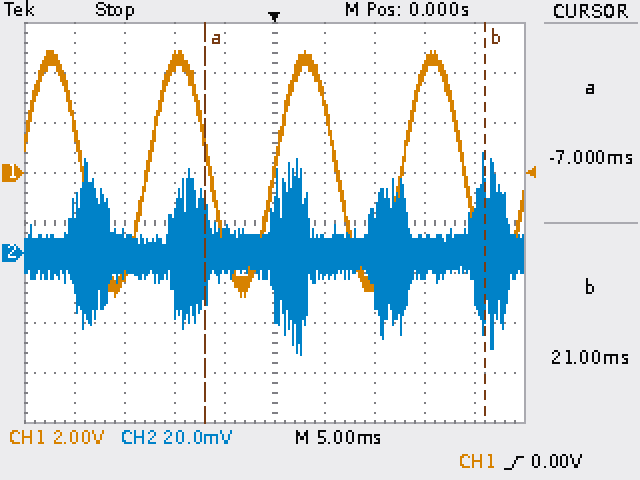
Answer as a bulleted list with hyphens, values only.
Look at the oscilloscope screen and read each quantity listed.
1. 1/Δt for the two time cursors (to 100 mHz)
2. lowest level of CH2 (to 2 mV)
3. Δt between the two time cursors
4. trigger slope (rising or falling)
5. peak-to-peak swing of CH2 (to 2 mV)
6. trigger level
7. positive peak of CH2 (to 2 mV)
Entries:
- 35.7 Hz
- -40 mV
- 28.0 ms
- rising
- 80 mV
- 0.00 V
- 40 mV
